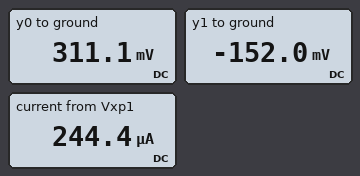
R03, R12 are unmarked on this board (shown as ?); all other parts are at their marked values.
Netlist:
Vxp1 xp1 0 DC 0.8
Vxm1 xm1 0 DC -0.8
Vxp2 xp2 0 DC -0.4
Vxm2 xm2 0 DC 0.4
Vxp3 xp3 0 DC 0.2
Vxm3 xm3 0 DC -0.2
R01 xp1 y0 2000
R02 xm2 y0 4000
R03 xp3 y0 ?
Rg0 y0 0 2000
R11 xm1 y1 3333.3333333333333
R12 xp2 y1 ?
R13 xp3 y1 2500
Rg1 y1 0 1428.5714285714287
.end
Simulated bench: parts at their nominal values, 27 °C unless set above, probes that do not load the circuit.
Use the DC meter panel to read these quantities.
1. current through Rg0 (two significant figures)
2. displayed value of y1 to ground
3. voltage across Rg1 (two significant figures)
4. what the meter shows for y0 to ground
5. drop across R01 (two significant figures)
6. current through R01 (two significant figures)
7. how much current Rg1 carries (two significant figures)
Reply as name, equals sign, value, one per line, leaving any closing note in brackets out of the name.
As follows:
current through Rg0 = 160 µA
displayed value of y1 to ground = -152.0 mV
voltage across Rg1 = 150 mV
what the meter shows for y0 to ground = 311.1 mV
drop across R01 = 490 mV
current through R01 = 240 µA
how much current Rg1 carries = 110 µA
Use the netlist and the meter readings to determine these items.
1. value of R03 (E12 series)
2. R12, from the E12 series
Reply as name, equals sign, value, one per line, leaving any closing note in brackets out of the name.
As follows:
value of R03 = 1 kΩ
R12, from the E12 series = 4.7 kΩ
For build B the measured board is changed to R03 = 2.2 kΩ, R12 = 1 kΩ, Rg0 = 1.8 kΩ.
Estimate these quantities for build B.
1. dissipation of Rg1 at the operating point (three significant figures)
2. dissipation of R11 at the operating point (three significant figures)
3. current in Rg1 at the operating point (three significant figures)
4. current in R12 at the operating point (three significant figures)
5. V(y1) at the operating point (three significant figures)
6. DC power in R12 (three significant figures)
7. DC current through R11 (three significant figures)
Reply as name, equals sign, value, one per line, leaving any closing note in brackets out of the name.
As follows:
dissipation of Rg1 at the operating point = 38.1 µW
dissipation of R11 at the operating point = 96.3 µW
current in Rg1 at the operating point = 163 µA
current in R12 at the operating point = 167 µA
V(y1) at the operating point = -233 mV
DC power in R12 = 27.8 µW
DC current through R11 = 170 µA
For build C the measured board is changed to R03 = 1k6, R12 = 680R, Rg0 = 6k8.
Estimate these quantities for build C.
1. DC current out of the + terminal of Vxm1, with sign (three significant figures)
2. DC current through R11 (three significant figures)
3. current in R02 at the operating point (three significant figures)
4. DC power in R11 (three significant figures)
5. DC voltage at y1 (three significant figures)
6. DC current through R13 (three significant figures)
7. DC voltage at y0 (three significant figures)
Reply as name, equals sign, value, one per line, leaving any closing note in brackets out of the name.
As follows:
DC current out of the + terminal of Vxm1, with sign = -162 µA
DC current through R11 = 162 µA
current in R02 at the operating point = 2.66 µA
DC power in R11 = 87.3 µW
DC voltage at y1 = -261 mV
DC current through R13 = 184 µA
DC voltage at y0 = 411 mV
